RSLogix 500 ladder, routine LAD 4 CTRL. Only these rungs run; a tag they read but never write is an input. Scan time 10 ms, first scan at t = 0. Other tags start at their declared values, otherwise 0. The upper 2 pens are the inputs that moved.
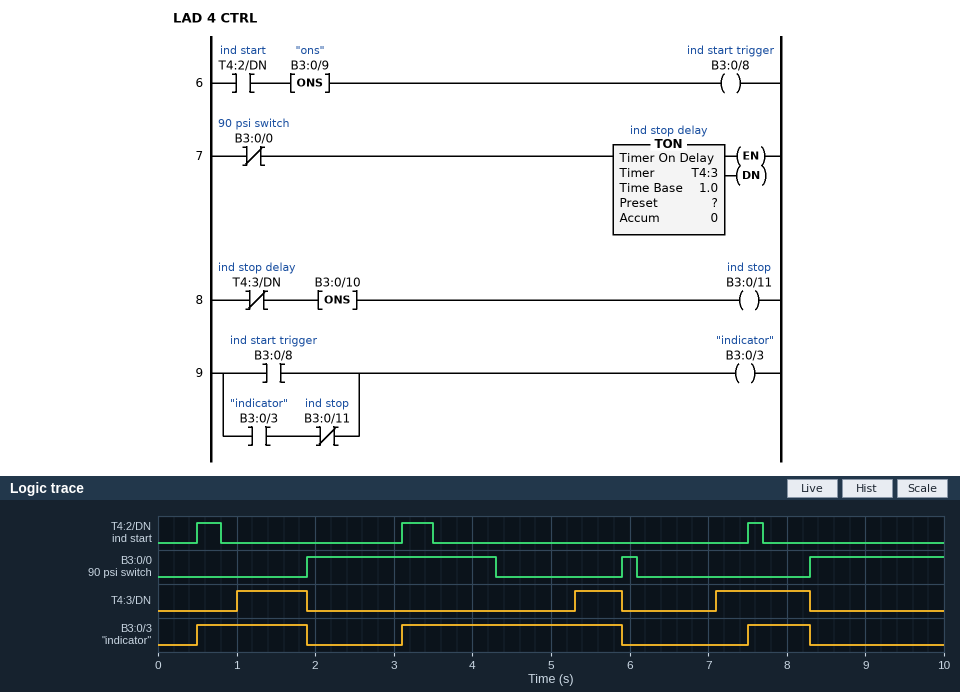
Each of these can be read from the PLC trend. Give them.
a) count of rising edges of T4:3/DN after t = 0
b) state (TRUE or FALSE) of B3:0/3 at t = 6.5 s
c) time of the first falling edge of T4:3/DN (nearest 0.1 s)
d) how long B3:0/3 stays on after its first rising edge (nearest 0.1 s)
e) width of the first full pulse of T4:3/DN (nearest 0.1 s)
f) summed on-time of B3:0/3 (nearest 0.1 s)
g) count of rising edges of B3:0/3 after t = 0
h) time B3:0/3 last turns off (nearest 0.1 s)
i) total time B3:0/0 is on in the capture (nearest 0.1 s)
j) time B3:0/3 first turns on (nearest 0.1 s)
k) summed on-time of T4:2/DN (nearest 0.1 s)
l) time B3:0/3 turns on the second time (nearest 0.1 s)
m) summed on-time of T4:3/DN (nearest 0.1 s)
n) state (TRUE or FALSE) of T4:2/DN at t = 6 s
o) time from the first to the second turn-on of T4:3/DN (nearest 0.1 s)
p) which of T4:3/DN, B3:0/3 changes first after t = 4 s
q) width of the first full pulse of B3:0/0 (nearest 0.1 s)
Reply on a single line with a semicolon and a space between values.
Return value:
3; FALSE; 1.9 s; 1.4 s; 0.9 s; 5.0 s; 3; 8.3 s; 4.3 s; 0.5 s; 0.9 s; 3.1 s; 2.7 s; FALSE; 4.3 s; T4:3/DN; 2.4 s
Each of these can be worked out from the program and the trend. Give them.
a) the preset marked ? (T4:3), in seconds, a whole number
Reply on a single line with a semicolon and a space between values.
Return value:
1 s
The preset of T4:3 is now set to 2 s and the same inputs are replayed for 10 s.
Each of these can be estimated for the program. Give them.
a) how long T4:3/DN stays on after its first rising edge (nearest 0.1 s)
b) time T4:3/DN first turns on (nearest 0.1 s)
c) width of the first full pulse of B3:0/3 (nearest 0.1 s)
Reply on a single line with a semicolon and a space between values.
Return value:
0.2 s; 8.1 s; 7.8 s
